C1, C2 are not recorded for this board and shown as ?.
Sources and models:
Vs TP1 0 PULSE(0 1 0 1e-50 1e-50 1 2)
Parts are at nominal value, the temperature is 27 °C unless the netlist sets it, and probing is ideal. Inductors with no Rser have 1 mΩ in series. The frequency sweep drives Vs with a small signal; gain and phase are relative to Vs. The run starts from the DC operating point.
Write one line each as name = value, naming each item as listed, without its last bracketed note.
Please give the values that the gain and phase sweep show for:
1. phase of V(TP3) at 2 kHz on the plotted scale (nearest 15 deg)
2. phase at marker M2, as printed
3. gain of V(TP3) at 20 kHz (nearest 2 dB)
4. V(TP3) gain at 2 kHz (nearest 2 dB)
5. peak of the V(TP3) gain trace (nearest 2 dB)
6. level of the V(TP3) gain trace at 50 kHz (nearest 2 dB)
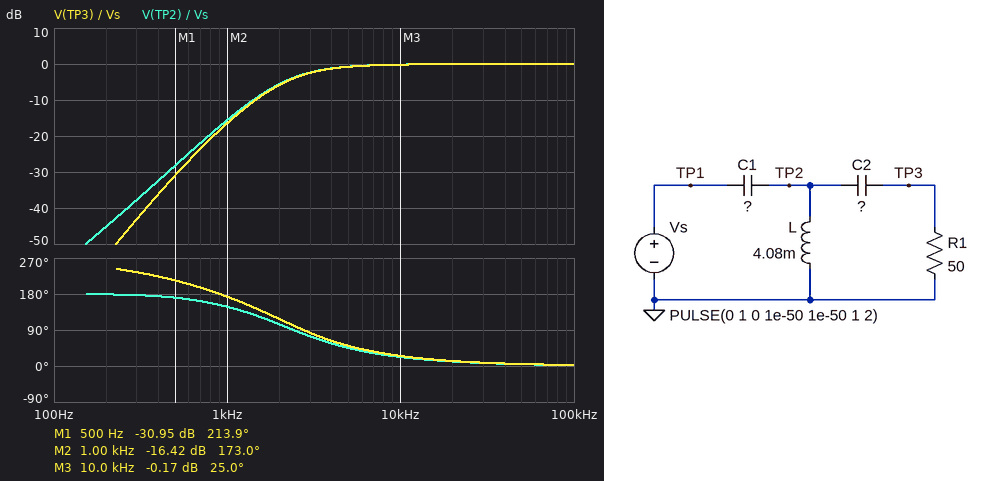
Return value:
phase of V(TP3) at 2 kHz on the plotted scale = 120 deg
phase at marker M2, as printed = 173.0 deg
gain of V(TP3) at 20 kHz = 0 dB
V(TP3) gain at 2 kHz = -6 dB
peak of the V(TP3) gain trace = 0 dB
level of the V(TP3) gain trace at 50 kHz = 0 dB
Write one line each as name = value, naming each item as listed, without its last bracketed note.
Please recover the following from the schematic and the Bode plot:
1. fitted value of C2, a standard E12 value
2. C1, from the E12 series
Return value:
fitted value of C2, a standard E12 value = 6.8 µF
C1, from the E12 series = 820 nF
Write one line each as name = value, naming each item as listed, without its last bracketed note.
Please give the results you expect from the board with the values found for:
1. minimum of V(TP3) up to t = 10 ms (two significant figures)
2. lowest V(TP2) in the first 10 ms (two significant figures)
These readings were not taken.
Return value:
minimum of V(TP3) up to t = 10 ms = -230 mV
lowest V(TP2) in the first 10 ms = -190 mV
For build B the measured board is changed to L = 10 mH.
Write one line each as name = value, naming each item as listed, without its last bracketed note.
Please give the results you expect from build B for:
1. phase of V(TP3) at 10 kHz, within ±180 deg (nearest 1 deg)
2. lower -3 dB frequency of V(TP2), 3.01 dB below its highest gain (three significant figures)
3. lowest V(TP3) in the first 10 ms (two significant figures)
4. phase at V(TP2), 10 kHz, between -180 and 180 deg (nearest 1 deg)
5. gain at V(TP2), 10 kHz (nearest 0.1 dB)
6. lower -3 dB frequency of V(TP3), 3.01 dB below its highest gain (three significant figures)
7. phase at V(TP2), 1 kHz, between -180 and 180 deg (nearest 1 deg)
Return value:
phase of V(TP3) at 10 kHz, within ±180 deg = 24 deg
lower -3 dB frequency of V(TP2), 3.01 dB below its highest gain = 3.47 kHz
lowest V(TP3) in the first 10 ms = -140 mV
phase at V(TP2), 10 kHz, between -180 and 180 deg = 21 deg
gain at V(TP2), 10 kHz = -0.5 dB
lower -3 dB frequency of V(TP3), 3.01 dB below its highest gain = 3.54 kHz
phase at V(TP2), 1 kHz, between -180 and 180 deg = 101 deg
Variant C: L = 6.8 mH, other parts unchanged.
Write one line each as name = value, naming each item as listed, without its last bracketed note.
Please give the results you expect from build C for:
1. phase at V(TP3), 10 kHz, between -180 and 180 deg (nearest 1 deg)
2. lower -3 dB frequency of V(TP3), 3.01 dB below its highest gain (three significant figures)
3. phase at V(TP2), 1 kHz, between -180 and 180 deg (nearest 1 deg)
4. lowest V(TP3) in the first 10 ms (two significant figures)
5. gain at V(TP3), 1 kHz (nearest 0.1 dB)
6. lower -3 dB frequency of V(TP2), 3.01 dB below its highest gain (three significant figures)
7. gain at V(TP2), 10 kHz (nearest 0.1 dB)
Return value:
phase at V(TP3), 10 kHz, between -180 and 180 deg = 24 deg
lower -3 dB frequency of V(TP3), 3.01 dB below its highest gain = 3.18 kHz
phase at V(TP2), 1 kHz, between -180 and 180 deg = 123 deg
lowest V(TP3) in the first 10 ms = -170 mV
gain at V(TP3), 1 kHz = -12.4 dB
lower -3 dB frequency of V(TP2), 3.01 dB below its highest gain = 3.11 kHz
gain at V(TP2), 10 kHz = -0.4 dB
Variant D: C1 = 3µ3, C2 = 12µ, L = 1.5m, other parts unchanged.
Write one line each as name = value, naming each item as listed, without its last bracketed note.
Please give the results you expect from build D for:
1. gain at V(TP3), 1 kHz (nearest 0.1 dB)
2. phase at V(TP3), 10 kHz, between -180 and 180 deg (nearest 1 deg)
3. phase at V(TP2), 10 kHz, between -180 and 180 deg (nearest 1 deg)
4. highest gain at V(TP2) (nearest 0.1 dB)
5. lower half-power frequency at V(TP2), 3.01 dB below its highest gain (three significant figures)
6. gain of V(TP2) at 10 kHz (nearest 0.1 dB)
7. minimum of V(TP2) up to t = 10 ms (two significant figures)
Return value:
gain at V(TP3), 1 kHz = -12.3 dB
phase at V(TP3), 10 kHz, between -180 and 180 deg = 7 deg
phase at V(TP2), 10 kHz, between -180 and 180 deg = 6 deg
highest gain at V(TP2) = 7.5 dB
lower half-power frequency at V(TP2), 3.01 dB below its highest gain = 1.91 kHz
gain of V(TP2) at 10 kHz = 0.4 dB
minimum of V(TP2) up to t = 10 ms = -550 mV
